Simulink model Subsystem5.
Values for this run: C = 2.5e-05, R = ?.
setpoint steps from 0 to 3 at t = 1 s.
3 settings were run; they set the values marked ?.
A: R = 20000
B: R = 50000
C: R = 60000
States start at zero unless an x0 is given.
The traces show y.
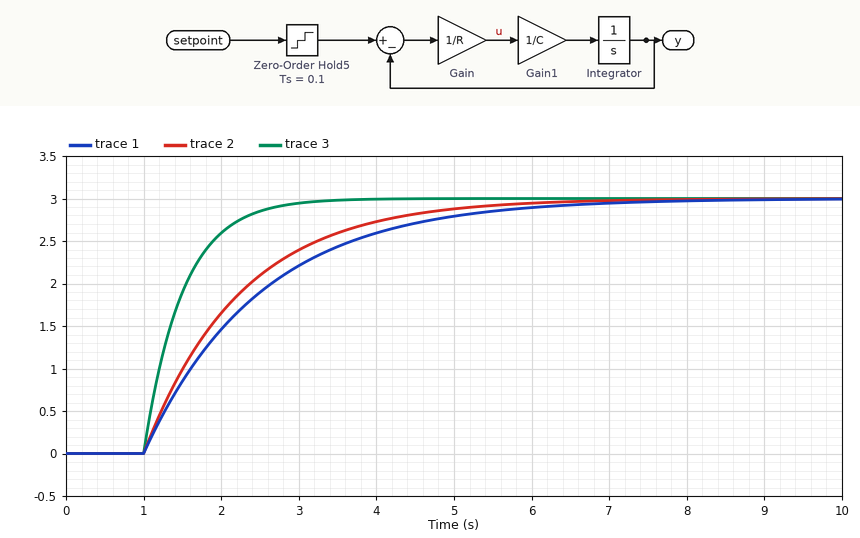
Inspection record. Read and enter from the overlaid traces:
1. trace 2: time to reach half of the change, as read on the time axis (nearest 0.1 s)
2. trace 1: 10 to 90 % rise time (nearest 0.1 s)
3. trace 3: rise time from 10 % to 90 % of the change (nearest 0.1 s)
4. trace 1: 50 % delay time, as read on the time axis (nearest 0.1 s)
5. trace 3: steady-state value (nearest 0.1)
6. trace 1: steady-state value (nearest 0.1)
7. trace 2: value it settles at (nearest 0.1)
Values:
1.9 s
3.3 s
1.1 s
2.0 s
3.0
3.0
3.0
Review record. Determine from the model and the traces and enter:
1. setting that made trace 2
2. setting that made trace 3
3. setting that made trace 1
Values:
B
A
C
